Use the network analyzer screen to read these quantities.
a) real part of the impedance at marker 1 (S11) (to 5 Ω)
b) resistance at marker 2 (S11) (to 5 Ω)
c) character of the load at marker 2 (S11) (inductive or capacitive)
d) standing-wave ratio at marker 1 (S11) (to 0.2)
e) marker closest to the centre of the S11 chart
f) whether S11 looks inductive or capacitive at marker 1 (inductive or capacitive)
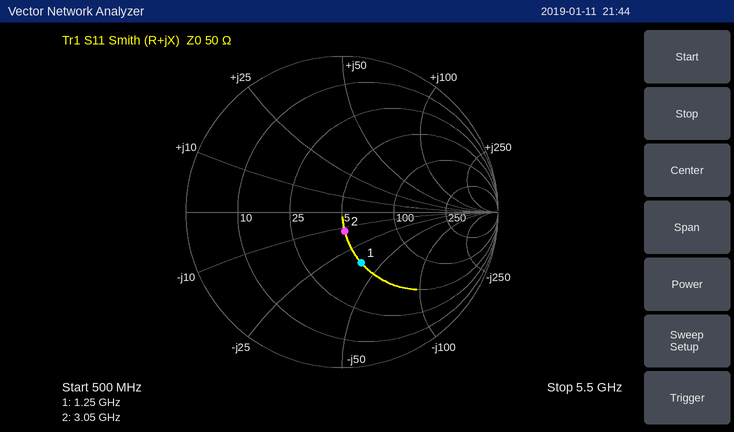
50 Ω
50 Ω
capacitive
2.0
marker 2
capacitive
